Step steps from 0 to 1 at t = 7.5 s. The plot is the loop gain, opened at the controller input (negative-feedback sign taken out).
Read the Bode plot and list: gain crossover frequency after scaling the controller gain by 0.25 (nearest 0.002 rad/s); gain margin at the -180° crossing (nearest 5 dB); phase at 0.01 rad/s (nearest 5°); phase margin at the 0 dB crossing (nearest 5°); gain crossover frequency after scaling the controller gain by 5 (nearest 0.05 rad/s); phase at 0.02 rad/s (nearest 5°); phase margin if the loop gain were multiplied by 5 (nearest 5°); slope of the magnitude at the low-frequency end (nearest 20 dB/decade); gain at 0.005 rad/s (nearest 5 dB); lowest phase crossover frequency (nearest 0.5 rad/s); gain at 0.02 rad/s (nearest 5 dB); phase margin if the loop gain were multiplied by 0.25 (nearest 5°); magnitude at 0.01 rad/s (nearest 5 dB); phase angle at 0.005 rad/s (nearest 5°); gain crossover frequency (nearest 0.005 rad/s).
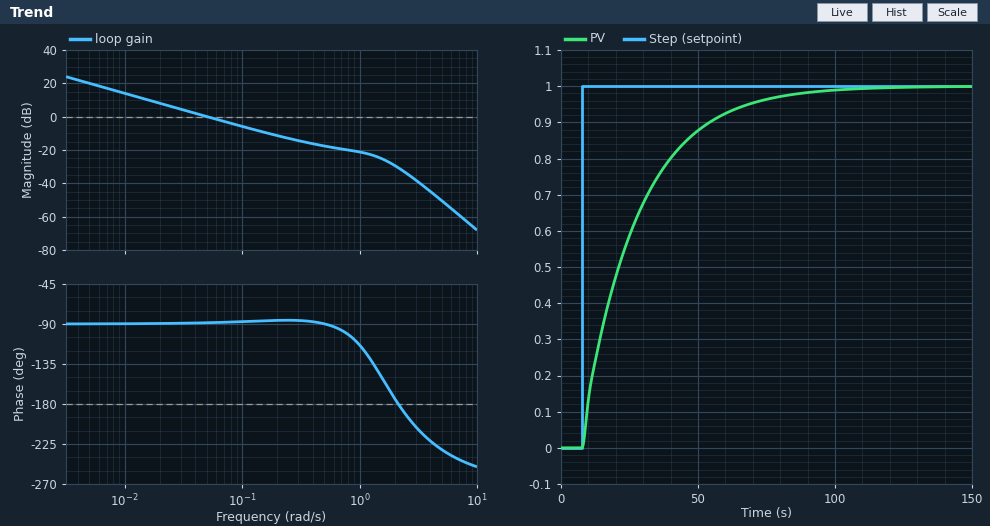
0.012 rad/s
30 dB
-90°
90°
0.30 rad/s
-90°
95°
-20 dB/decade
20 dB
2.0 rad/s
10 dB
90°
15 dB
-90°
0.050 rad/s
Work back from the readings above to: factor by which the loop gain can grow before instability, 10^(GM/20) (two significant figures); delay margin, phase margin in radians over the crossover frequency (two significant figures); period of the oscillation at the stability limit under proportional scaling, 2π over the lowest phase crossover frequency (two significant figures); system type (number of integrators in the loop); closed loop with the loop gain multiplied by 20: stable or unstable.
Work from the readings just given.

32
31 s
3.1 s
1
stable
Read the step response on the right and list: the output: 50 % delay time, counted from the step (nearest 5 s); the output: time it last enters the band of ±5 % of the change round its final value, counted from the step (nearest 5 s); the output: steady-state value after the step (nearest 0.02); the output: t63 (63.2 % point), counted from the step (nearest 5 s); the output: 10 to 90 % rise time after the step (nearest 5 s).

15 s
60 s
1.00
20 s
45 s
